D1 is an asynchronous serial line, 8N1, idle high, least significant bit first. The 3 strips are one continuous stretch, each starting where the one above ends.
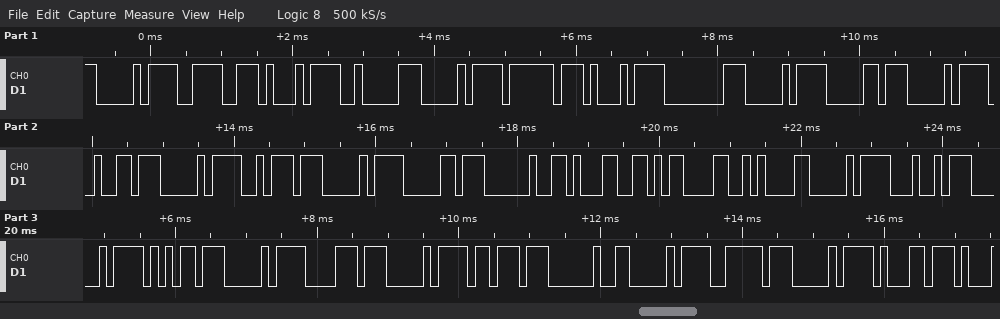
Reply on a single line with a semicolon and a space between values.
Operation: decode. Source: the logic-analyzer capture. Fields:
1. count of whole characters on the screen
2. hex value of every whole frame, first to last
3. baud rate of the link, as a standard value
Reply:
33; D0 9E D1 82 D0 BF D1 80 D0 B0 D0 B2 D0 BA D0 B0 20 31 0D 0A D0 A4 D0 B5 D0 B8 D0 BB 20 D0 BE D0 B1; 9600 baud
